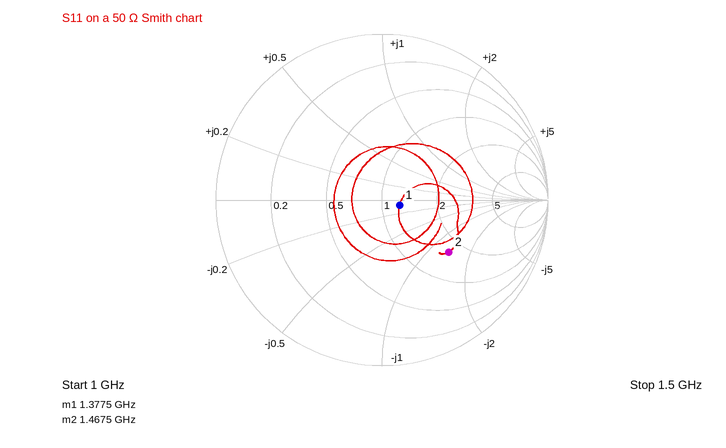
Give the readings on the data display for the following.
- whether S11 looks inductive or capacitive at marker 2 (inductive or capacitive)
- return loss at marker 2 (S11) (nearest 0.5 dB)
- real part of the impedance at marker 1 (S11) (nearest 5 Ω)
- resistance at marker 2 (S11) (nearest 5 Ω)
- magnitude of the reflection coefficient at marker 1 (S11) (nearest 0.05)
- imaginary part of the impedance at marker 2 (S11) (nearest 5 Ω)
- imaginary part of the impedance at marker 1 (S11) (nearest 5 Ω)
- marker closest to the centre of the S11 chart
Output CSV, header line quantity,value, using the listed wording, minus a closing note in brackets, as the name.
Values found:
quantity,value
whether S11 looks inductive or capacitive at marker 2,capacitive
return loss at marker 2 (S11),6.0 dB
real part of the impedance at marker 1 (S11),60 Ω
resistance at marker 2 (S11),80 Ω
magnitude of the reflection coefficient at marker 1 (S11),0.10
imaginary part of the impedance at marker 2 (S11),-70 Ω
imaginary part of the impedance at marker 1 (S11),-5 Ω
marker closest to the centre of the S11 chart,marker 1
